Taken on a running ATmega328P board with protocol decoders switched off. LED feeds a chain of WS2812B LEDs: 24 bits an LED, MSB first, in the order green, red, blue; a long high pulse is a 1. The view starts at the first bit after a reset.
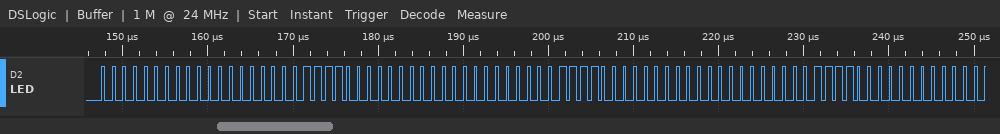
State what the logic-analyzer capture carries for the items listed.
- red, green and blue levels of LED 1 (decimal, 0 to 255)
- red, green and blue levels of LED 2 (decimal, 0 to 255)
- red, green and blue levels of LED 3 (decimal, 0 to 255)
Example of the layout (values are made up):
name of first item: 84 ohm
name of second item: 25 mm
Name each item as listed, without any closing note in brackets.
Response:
red, green and blue levels of LED 1: 0, 0, 30
red, green and blue levels of LED 2: 0, 0, 30
red, green and blue levels of LED 3: 0, 0, 30
